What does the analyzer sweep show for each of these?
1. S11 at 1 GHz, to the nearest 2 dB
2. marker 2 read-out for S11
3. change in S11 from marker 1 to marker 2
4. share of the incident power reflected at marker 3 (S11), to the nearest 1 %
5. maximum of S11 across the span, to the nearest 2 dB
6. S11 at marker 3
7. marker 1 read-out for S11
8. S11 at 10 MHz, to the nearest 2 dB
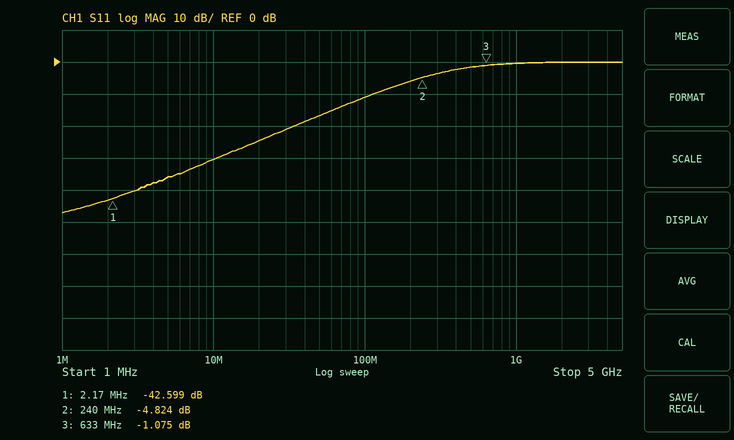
0 dB
-4.824 dB
37.775 dB
78 %
0 dB
-1.075 dB
-42.599 dB
-30 dB
